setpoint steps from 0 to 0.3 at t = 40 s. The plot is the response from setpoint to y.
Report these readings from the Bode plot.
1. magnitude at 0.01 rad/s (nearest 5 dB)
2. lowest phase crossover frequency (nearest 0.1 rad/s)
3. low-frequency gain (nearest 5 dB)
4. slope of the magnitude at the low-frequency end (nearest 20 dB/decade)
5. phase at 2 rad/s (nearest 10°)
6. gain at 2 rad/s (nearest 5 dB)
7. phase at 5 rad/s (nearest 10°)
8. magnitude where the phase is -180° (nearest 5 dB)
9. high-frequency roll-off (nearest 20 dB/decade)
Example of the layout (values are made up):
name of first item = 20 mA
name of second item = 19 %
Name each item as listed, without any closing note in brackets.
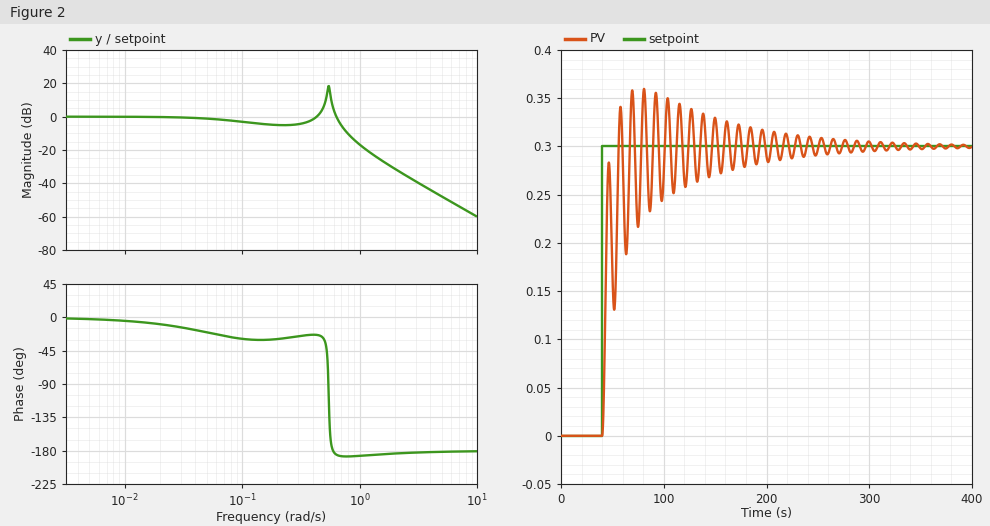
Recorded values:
magnitude at 0.01 rad/s = 0 dB
lowest phase crossover frequency = 0.6 rad/s
low-frequency gain = 0 dB
slope of the magnitude at the low-frequency end = 0 dB/decade
phase at 2 rad/s = -180°
gain at 2 rad/s = -30 dB
phase at 5 rad/s = -180°
magnitude where the phase is -180° = 5 dB
high-frequency roll-off = -40 dB/decade
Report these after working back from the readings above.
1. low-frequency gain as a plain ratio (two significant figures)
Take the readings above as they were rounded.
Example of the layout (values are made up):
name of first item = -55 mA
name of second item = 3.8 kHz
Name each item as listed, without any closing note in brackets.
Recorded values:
low-frequency gain as a plain ratio = 1.0
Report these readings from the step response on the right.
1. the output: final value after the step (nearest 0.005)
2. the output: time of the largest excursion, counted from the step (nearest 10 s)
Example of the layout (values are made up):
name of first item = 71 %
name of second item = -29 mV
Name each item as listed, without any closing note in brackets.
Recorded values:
the output: final value after the step = 0.300
the output: time of the largest excursion, counted from the step = 40 s
